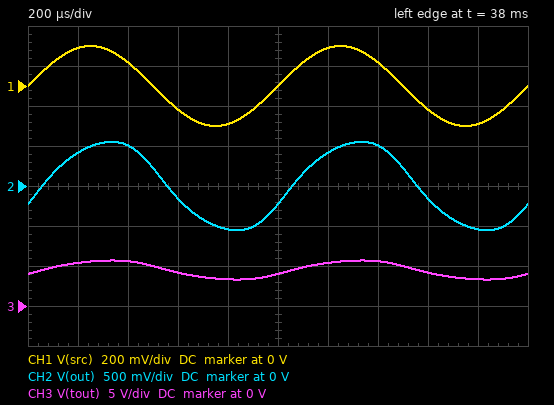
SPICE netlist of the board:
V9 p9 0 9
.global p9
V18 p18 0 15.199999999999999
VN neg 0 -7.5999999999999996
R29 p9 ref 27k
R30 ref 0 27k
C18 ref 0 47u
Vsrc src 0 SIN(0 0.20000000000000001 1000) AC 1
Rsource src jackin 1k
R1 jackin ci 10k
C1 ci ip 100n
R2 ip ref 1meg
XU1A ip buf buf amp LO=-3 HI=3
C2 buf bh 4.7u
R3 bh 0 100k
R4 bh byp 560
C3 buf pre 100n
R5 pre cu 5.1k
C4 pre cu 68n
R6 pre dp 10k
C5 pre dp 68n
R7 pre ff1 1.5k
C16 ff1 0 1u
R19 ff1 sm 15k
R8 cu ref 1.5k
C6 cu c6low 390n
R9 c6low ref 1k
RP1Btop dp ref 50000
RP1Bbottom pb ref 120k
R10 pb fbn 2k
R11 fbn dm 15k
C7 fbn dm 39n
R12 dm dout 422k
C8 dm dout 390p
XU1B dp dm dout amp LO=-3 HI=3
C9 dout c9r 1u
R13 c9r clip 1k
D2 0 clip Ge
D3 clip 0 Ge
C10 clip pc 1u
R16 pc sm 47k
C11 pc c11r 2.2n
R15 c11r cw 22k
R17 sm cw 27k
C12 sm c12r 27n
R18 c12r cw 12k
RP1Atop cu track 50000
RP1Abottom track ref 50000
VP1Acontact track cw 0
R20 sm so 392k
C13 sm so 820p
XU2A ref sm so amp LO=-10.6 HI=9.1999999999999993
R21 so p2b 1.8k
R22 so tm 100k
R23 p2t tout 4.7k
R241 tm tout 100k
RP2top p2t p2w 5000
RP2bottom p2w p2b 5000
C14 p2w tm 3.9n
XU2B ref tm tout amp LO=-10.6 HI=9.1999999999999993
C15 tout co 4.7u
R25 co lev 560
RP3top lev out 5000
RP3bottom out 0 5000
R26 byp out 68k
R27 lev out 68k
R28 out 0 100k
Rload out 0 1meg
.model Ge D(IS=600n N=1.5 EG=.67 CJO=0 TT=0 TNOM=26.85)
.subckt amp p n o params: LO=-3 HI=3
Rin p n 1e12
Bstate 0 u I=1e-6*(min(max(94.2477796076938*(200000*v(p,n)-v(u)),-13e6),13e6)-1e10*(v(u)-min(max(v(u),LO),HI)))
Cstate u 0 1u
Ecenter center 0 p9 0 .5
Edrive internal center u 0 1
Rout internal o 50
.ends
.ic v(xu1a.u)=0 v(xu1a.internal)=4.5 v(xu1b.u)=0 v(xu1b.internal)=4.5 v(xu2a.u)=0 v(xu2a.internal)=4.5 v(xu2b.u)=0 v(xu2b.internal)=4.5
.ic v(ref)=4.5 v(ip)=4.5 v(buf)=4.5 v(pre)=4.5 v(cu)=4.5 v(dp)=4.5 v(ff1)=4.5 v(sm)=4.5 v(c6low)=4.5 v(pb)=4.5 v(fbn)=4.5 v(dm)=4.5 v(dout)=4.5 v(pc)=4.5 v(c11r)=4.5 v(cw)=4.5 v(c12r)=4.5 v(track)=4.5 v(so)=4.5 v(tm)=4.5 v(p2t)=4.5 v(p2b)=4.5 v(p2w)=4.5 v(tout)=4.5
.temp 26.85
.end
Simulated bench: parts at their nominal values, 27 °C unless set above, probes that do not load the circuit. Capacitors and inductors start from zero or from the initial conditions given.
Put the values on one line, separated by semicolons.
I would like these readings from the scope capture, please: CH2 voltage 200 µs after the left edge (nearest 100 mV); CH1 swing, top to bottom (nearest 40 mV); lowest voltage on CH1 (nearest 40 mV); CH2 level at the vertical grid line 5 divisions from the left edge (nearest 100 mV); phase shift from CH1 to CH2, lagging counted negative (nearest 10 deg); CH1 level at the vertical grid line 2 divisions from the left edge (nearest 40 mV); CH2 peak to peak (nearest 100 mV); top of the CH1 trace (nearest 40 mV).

400 mV; 400 mV; -200 mV; -200 mV; -20 deg; 120 mV; 1.1 V; 200 mV
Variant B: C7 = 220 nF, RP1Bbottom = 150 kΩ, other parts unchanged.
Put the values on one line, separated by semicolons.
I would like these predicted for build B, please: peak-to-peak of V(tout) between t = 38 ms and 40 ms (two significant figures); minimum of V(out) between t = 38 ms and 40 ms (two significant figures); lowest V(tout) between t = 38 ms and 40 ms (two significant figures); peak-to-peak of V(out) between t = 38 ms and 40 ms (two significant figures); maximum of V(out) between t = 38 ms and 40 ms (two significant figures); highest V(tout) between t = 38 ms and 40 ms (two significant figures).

2.2 V; -510 mV; 3.4 V; 1.0 V; 510 mV; 5.6 V
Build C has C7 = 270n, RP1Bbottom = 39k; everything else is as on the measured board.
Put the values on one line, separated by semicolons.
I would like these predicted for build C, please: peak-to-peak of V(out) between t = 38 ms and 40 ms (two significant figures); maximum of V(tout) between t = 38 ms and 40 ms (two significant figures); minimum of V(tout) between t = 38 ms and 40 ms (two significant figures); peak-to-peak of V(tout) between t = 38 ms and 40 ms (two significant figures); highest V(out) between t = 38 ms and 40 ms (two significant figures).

1.5 V; 6.1 V; 2.9 V; 3.3 V; 750 mV
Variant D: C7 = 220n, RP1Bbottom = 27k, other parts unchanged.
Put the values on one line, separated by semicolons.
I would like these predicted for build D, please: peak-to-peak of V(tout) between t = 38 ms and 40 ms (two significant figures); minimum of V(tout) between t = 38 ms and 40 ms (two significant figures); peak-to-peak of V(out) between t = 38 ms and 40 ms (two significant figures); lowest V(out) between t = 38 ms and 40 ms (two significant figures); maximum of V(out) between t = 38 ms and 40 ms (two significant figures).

3.5 V; 2.7 V; 1.6 V; -810 mV; 810 mV
